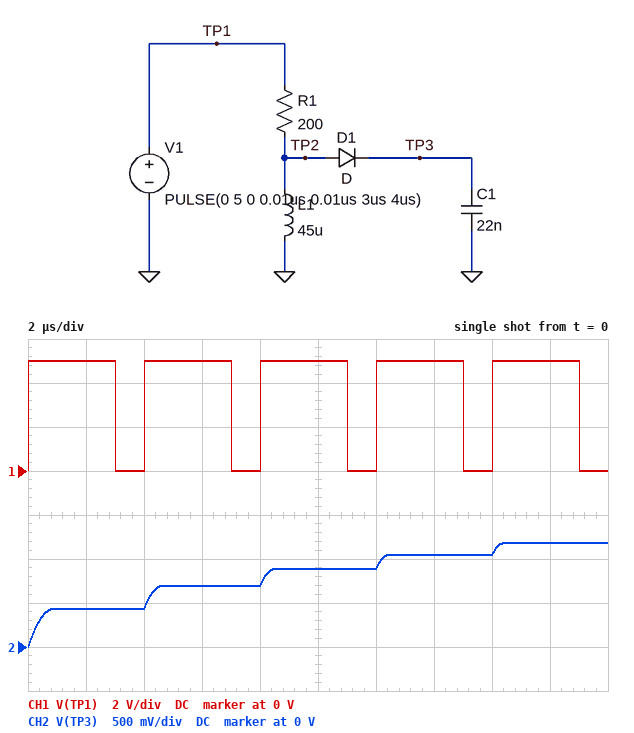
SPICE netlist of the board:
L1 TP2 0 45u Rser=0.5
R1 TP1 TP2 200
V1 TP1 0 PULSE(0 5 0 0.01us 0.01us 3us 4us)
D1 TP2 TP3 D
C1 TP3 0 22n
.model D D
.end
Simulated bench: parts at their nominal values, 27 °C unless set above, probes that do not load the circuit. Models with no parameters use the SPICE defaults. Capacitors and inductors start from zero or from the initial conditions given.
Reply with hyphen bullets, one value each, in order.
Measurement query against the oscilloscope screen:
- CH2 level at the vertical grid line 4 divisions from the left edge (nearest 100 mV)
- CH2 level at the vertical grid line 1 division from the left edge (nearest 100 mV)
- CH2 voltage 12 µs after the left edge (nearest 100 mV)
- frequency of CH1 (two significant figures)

- 700 mV
- 400 mV
- 900 mV
- 250 kHz
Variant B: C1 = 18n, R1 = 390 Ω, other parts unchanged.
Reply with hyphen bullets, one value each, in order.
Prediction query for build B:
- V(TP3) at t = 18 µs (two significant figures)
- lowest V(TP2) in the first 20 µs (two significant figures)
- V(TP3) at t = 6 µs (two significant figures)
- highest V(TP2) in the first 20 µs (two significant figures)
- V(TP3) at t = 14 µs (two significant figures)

- 620 mV
- -4.8 V
- 320 mV
- 1.3 V
- 530 mV
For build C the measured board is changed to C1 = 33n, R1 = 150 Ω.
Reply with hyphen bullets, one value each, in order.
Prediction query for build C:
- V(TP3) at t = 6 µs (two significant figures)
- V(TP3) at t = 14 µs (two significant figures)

- 750 mV
- 1.1 V
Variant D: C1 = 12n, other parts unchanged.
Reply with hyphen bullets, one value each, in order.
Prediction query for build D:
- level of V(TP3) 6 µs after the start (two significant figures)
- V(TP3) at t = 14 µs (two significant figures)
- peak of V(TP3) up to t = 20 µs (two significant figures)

- 990 mV
- 1.4 V
- 1.6 V
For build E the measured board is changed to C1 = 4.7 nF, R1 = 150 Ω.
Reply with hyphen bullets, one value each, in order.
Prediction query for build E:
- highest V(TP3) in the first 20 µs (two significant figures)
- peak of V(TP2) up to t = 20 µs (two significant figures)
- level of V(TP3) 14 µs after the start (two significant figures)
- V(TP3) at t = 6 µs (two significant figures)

- 2.6 V
- 3.3 V
- 2.4 V
- 1.9 V
